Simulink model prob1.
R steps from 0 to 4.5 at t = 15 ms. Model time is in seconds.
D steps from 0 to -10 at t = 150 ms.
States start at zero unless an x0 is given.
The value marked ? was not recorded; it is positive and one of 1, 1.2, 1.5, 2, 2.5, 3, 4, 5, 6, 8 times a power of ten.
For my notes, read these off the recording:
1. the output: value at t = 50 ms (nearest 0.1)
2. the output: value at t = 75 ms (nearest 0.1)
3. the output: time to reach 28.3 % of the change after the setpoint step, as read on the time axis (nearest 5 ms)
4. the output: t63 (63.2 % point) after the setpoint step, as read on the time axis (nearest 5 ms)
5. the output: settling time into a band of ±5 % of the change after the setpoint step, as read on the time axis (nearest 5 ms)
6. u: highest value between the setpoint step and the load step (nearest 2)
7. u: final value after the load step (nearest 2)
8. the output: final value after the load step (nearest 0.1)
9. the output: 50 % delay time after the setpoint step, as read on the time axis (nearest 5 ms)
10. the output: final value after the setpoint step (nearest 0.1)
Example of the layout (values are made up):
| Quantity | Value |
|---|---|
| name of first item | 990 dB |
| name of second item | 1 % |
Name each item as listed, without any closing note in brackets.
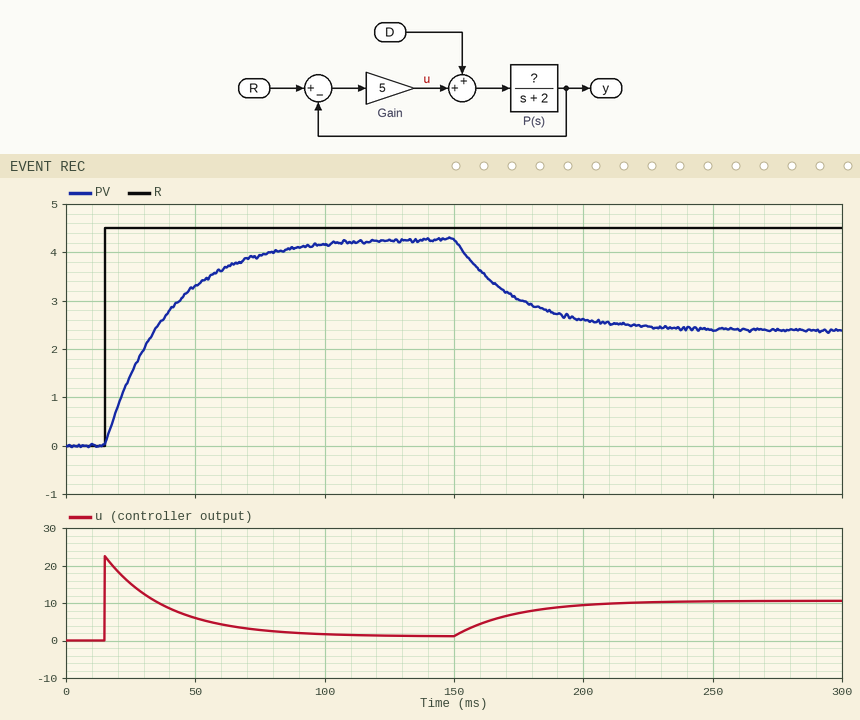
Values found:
| Quantity | Value |
|---|---|
| the output: value at t = 50 ms | 3.3 |
| the output: value at t = 75 ms | 3.9 |
| the output: time to reach 28.3 % of the change after the setpoint step, as read on the time axis | 25 ms |
| the output: t63 (63.2 % point) after the setpoint step, as read on the time axis | 40 ms |
| the output: settling time into a band of ±5 % of the change after the setpoint step, as read on the time axis | 85 ms |
| u: highest value between the setpoint step and the load step | 22 |
| u: final value after the load step | 10 |
| the output: final value after the load step | 2.4 |
| the output: 50 % delay time after the setpoint step, as read on the time axis | 30 ms |
| the output: final value after the setpoint step | 4.3 |
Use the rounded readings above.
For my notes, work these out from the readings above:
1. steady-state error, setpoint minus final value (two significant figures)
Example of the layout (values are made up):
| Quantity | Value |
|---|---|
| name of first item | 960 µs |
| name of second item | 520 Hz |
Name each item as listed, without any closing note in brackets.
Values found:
| Quantity | Value |
|---|---|
| steady-state error, setpoint minus final value | 0.20 |
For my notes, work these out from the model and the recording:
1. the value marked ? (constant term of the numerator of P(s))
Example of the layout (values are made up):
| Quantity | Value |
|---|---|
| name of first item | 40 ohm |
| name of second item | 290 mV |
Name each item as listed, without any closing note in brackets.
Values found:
| Quantity | Value |
|---|---|
| the value marked ? (constant term of the numerator of P(s)) | 8 |
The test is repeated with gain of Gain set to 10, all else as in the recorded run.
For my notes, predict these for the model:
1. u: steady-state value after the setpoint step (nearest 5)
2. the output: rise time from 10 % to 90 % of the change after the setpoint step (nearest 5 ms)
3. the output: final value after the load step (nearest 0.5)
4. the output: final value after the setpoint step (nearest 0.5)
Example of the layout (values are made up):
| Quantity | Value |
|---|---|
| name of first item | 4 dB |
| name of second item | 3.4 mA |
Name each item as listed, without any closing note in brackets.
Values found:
| Quantity | Value |
|---|---|
| u: steady-state value after the setpoint step | 0 |
| the output: rise time from 10 % to 90 % of the change after the setpoint step | 25 ms |
| the output: final value after the load step | 3.5 |
| the output: final value after the setpoint step | 4.5 |
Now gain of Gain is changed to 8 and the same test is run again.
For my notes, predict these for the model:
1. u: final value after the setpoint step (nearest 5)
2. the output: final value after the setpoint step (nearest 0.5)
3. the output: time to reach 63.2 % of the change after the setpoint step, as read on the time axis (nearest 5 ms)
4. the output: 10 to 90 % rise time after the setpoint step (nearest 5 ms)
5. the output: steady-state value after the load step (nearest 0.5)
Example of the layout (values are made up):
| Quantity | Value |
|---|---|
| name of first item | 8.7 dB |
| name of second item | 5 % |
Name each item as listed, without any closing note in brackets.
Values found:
| Quantity | Value |
|---|---|
| u: final value after the setpoint step | 0 |
| the output: final value after the setpoint step | 4.5 |
| the output: time to reach 63.2 % of the change after the setpoint step, as read on the time axis | 30 ms |
| the output: 10 to 90 % rise time after the setpoint step | 35 ms |
| the output: steady-state value after the load step | 3.0 |
